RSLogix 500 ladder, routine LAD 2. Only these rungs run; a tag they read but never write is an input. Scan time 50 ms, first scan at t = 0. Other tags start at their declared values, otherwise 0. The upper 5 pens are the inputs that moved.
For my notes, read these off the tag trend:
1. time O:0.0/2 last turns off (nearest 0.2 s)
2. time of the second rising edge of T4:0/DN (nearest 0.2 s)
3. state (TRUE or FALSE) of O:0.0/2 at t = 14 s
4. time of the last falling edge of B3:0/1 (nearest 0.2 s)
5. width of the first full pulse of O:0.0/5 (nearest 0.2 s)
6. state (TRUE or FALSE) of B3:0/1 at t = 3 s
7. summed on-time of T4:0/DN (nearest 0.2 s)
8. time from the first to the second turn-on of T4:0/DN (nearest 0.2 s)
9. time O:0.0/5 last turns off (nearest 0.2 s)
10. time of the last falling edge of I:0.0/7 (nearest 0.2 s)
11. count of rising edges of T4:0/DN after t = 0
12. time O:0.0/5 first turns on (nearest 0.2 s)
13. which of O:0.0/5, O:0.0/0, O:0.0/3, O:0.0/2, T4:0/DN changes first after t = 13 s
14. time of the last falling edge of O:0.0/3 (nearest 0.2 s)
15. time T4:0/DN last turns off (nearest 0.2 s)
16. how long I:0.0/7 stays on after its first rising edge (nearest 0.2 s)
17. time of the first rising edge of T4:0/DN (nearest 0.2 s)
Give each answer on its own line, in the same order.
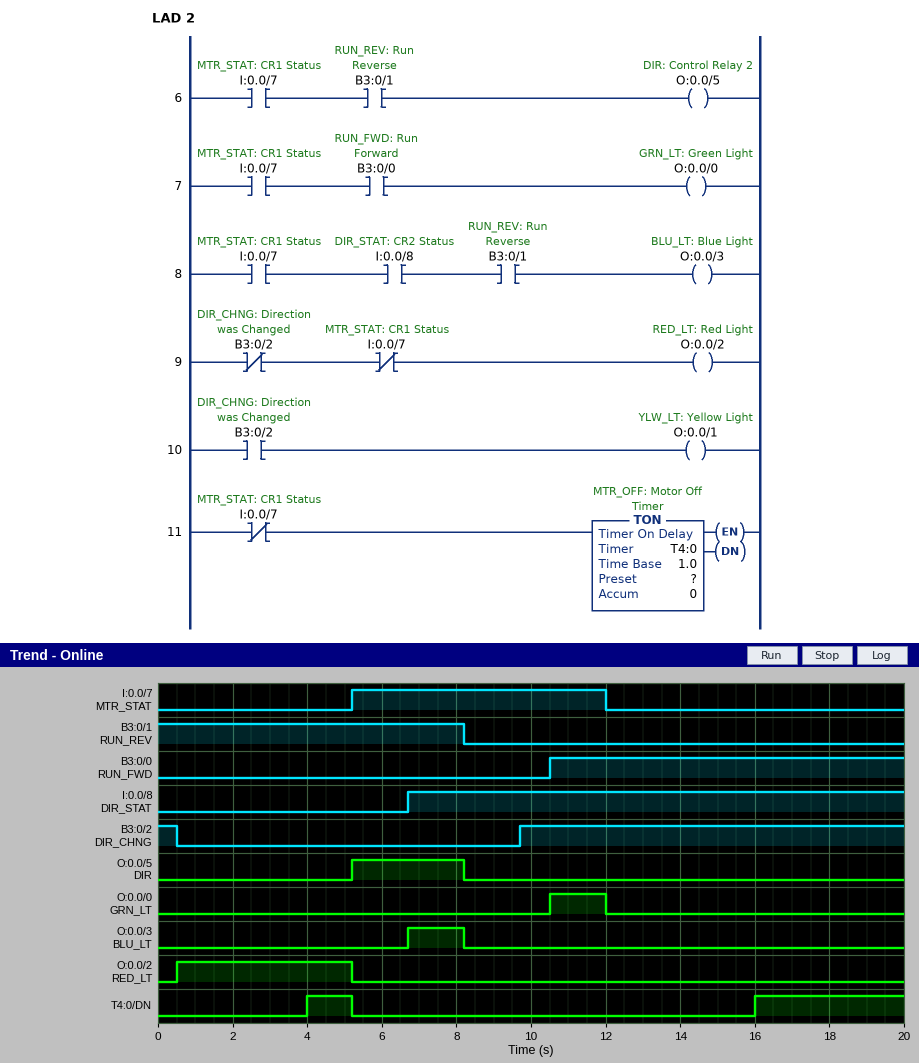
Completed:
5.2 s
16.0 s
FALSE
8.2 s
3.0 s
TRUE
5.2 s
12.0 s
8.2 s
12.0 s
2
5.2 s
T4:0/DN
8.2 s
5.2 s
6.8 s
4.0 s
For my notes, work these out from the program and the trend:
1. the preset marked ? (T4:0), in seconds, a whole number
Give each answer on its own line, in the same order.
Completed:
4 s
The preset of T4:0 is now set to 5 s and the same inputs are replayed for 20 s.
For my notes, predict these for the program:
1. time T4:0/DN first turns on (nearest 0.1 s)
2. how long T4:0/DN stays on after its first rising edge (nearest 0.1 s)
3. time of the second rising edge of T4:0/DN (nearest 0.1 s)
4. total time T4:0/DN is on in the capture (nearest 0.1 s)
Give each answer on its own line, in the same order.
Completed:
5.0 s
0.2 s
17.0 s
3.2 s
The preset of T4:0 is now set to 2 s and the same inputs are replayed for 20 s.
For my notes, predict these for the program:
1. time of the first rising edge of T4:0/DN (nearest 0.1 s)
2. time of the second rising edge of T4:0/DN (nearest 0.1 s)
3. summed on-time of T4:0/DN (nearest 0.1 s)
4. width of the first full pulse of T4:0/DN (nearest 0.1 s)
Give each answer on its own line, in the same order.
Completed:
2.0 s
14.0 s
9.2 s
3.2 s
